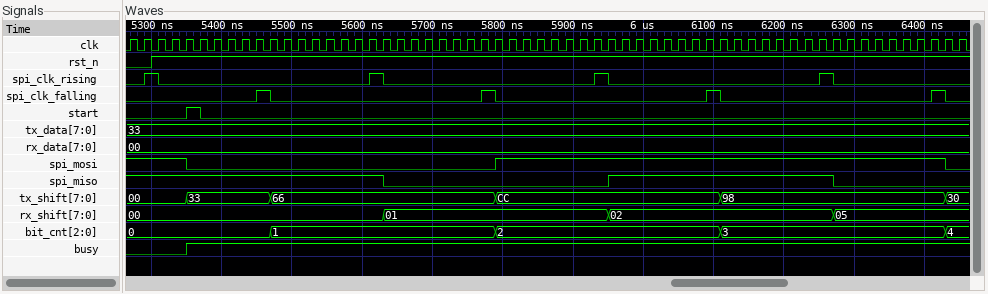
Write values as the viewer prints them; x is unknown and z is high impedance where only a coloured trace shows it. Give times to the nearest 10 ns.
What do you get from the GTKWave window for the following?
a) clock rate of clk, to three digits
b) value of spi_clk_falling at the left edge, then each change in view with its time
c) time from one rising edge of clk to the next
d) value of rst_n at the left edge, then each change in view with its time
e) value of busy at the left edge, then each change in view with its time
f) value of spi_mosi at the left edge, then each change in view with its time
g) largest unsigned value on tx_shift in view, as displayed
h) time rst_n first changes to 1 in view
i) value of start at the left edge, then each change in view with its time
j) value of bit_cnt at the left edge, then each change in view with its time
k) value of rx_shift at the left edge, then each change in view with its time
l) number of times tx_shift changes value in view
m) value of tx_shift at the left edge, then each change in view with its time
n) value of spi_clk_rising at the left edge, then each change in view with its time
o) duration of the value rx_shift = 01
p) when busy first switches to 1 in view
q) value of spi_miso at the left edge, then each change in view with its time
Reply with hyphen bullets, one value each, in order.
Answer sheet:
- 50.0 MHz
- 0, 1 at 5450 ns, 0 at 5470 ns, 1 at 5770 ns, 0 at 5790 ns, 1 at 6090 ns, 0 at 6110 ns, 1 at 6410 ns, 0 at 6430 ns
- 20 ns
- 0, 1 at 5300 ns
- 0, 1 at 5350 ns
- 1, 0 at 5350 ns, 1 at 5790 ns, 0 at 6430 ns
- CC
- 5300 ns
- 0, 1 at 5350 ns, 0 at 5370 ns
- 0, 1 at 5470 ns, 2 at 5790 ns, 3 at 6110 ns, 4 at 6430 ns
- 00, 01 at 5630 ns, 02 at 5950 ns, 05 at 6270 ns
- 5
- 00, 33 at 5350 ns, 66 at 5470 ns, CC at 5790 ns, 98 at 6110 ns, 30 at 6430 ns
- 0, 1 at 5290 ns, 0 at 5310 ns, 1 at 5610 ns, 0 at 5630 ns, 1 at 5930 ns, 0 at 5950 ns, 1 at 6250 ns, 0 at 6270 ns
- 320 ns
- 5350 ns
- 1, 0 at 5630 ns, 1 at 5950 ns, 0 at 6270 ns
